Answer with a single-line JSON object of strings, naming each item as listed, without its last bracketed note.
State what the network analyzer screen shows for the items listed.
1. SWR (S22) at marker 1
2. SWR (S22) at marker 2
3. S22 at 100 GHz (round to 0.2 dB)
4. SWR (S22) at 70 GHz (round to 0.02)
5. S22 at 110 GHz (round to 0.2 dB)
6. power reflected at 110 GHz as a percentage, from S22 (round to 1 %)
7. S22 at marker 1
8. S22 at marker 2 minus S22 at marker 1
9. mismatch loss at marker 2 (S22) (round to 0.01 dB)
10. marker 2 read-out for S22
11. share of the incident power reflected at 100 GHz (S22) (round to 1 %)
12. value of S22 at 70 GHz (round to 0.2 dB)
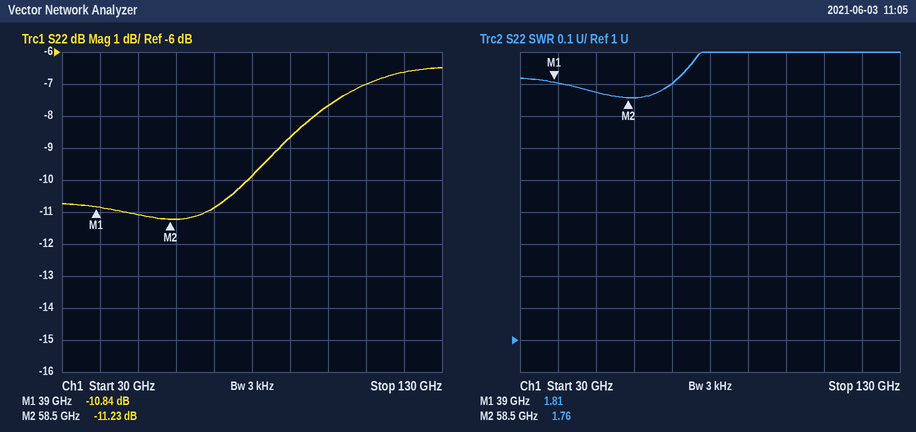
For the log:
{"SWR (S22) at marker 1": "1.81", "SWR (S22) at marker 2": "1.76", "S22 at 100 GHz": "-7.6 dB", "SWR (S22) at 70 GHz": "1.80", "S22 at 110 GHz": "-7.0 dB", "power reflected at 110 GHz as a percentage, from S22": "20 %", "S22 at marker 1": "-10.84 dB", "S22 at marker 2 minus S22 at marker 1": "-0.39 dB", "mismatch loss at marker 2 (S22)": "0.34 dB", "marker 2 read-out for S22": "-11.23 dB", "share of the incident power reflected at 100 GHz (S22)": "17 %", "value of S22 at 70 GHz": "-10.8 dB"}
